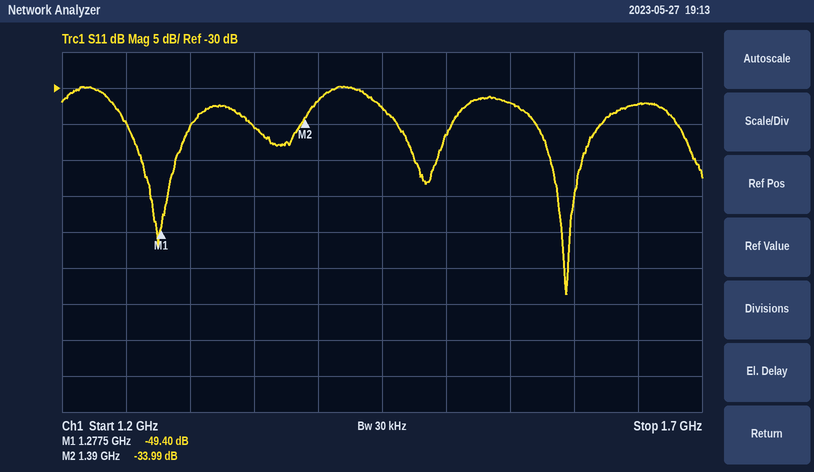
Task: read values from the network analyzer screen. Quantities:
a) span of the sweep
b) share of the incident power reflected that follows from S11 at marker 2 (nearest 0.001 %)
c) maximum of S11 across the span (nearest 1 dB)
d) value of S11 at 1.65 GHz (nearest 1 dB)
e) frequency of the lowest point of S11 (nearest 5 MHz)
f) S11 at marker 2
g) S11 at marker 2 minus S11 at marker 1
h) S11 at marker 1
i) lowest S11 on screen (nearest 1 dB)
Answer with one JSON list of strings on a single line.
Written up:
["500 MHz", "0.040 %", "-30 dB", "-32 dB", "1.595 GHz", "-33.99 dB", "15.41 dB", "-49.40 dB", "-59 dB"]
